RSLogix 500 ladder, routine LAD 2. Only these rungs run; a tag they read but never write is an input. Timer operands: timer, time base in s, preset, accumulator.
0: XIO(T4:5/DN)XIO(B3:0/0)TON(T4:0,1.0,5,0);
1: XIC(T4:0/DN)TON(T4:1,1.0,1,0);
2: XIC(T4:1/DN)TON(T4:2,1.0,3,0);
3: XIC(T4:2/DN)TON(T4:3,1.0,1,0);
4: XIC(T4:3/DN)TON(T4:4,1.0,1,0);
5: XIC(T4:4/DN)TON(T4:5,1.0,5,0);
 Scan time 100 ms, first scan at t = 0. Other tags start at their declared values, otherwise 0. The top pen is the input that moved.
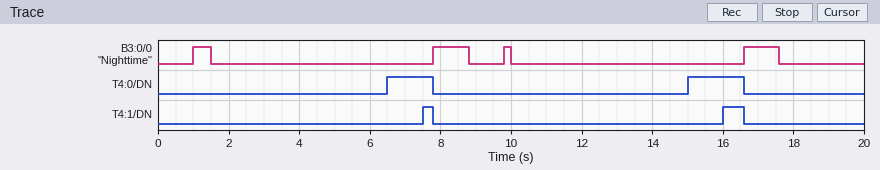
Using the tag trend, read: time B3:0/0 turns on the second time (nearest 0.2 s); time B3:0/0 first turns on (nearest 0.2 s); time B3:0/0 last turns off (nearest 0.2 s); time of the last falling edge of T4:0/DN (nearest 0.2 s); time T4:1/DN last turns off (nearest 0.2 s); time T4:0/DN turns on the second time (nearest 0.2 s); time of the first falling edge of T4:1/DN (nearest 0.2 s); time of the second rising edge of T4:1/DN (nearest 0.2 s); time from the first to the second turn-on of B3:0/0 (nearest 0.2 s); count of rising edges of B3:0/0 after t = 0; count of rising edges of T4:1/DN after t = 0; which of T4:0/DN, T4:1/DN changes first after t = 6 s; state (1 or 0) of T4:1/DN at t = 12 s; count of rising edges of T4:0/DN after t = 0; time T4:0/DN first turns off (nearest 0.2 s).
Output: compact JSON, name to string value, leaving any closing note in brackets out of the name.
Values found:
{"time B3:0/0 turns on the second time": "7.8 s", "time B3:0/0 first turns on": "1.0 s", "time B3:0/0 last turns off": "17.6 s", "time of the last falling edge of T4:0/DN": "16.6 s", "time T4:1/DN last turns off": "16.6 s", "time T4:0/DN turns on the second time": "15.0 s", "time of the first falling edge of T4:1/DN": "7.8 s", "time of the second rising edge of T4:1/DN": "16.0 s", "time from the first to the second turn-on of B3:0/0": "6.8 s", "count of rising edges of B3:0/0 after t = 0": "4", "count of rising edges of T4:1/DN after t = 0": "2", "which of T4:0/DN, T4:1/DN changes first after t = 6 s": "T4:0/DN", "state (1 or 0) of T4:1/DN at t = 12 s": "0", "count of rising edges of T4:0/DN after t = 0": "2", "time T4:0/DN first turns off": "7.8 s"}
